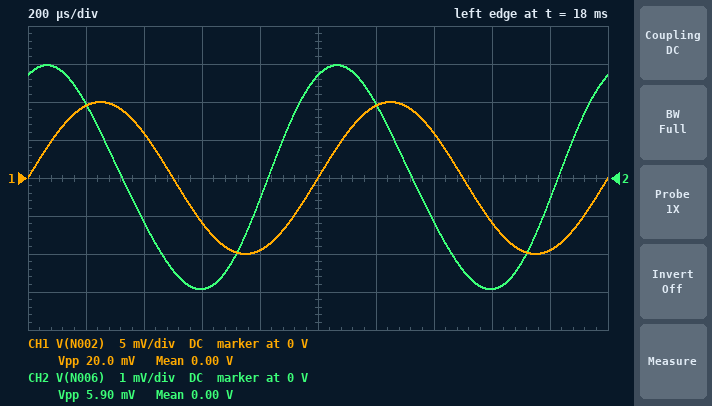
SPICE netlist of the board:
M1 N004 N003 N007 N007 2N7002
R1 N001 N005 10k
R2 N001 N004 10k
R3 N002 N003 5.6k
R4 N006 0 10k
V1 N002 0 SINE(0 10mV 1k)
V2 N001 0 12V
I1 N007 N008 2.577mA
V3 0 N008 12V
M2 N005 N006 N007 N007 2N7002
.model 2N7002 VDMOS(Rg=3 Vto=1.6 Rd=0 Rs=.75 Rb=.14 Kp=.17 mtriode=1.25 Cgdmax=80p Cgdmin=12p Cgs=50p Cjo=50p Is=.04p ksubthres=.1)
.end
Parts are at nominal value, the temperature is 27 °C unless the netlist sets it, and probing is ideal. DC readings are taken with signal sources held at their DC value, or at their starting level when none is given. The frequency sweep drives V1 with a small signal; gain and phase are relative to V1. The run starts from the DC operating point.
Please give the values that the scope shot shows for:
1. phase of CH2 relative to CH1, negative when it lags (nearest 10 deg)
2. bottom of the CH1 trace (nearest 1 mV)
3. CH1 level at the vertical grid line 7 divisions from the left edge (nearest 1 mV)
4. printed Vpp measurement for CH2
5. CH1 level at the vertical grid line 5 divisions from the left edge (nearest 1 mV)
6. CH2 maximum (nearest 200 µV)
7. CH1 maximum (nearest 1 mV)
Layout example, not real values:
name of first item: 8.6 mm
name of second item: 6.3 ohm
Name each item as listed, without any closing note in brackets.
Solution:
phase of CH2 relative to CH1, negative when it lags: 60 deg
bottom of the CH1 trace: -10 mV
CH1 level at the vertical grid line 7 divisions from the left edge: 6 mV
printed Vpp measurement for CH2: 5.90 mV
CH1 level at the vertical grid line 5 divisions from the left edge: 0 V
CH2 maximum: 3.0 mV
CH1 maximum: 10 mV
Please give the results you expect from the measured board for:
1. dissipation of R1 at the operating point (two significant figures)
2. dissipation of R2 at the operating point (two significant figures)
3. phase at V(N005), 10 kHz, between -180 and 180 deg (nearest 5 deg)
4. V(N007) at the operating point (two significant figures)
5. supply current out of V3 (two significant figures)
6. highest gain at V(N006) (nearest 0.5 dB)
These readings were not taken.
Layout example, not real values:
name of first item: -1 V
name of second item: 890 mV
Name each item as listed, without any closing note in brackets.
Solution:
dissipation of R1 at the operating point: 17 mW
dissipation of R2 at the operating point: 17 mW
phase at V(N005), 10 kHz, between -180 and 180 deg: -80 deg
V(N007) at the operating point: -1.7 V
supply current out of V3: 2.6 mA
highest gain at V(N006): -4.0 dB
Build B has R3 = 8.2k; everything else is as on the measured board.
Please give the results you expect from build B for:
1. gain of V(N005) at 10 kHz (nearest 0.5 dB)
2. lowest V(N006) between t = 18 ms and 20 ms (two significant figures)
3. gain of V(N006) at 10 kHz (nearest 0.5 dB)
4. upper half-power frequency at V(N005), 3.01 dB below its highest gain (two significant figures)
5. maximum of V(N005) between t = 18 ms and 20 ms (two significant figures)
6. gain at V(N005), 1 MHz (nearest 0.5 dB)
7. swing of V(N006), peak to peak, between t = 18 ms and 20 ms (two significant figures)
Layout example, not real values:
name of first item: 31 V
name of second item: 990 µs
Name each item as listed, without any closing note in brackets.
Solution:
gain of V(N005) at 10 kHz: 21.5 dB
lowest V(N006) between t = 18 ms and 20 ms: -2.8 mV
gain of V(N006) at 10 kHz: -5.5 dB
upper half-power frequency at V(N005), 3.01 dB below its highest gain: 1.6 kHz
maximum of V(N005) between t = 18 ms and 20 ms: -260 mV
gain at V(N005), 1 MHz: -10.5 dB
swing of V(N006), peak to peak, between t = 18 ms and 20 ms: 5.7 mV
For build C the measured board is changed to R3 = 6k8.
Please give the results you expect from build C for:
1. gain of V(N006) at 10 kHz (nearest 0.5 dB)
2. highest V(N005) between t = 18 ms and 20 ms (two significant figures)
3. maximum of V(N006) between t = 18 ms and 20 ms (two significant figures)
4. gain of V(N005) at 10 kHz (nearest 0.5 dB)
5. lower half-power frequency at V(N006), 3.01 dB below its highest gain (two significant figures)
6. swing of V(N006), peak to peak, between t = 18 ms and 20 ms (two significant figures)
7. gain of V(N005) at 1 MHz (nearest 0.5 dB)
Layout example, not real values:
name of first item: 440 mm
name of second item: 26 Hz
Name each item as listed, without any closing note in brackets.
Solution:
gain of V(N006) at 10 kHz: -5.0 dB
highest V(N005) between t = 18 ms and 20 ms: -240 mV
maximum of V(N006) between t = 18 ms and 20 ms: 2.9 mV
gain of V(N005) at 10 kHz: 22.0 dB
lower half-power frequency at V(N006), 3.01 dB below its highest gain: 1.7 kHz
swing of V(N006), peak to peak, between t = 18 ms and 20 ms: 5.8 mV
gain of V(N005) at 1 MHz: -9.5 dB
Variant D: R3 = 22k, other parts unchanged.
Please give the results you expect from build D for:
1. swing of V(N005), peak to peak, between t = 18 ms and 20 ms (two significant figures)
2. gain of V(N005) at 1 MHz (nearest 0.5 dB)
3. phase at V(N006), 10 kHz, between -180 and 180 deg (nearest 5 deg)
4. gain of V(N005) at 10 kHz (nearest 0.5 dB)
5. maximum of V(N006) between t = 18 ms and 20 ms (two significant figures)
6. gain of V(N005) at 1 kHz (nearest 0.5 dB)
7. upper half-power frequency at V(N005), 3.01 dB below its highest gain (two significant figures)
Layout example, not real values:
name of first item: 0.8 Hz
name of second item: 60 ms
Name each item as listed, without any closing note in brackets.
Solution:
swing of V(N005), peak to peak, between t = 18 ms and 20 ms: 1.0 V
gain of V(N005) at 1 MHz: -17.5 dB
phase at V(N006), 10 kHz, between -180 and 180 deg: 0 deg
gain of V(N005) at 10 kHz: 16.5 dB
maximum of V(N006) between t = 18 ms and 20 ms: 2.3 mV
gain of V(N005) at 1 kHz: 34.0 dB
upper half-power frequency at V(N005), 3.01 dB below its highest gain: 920 Hz
